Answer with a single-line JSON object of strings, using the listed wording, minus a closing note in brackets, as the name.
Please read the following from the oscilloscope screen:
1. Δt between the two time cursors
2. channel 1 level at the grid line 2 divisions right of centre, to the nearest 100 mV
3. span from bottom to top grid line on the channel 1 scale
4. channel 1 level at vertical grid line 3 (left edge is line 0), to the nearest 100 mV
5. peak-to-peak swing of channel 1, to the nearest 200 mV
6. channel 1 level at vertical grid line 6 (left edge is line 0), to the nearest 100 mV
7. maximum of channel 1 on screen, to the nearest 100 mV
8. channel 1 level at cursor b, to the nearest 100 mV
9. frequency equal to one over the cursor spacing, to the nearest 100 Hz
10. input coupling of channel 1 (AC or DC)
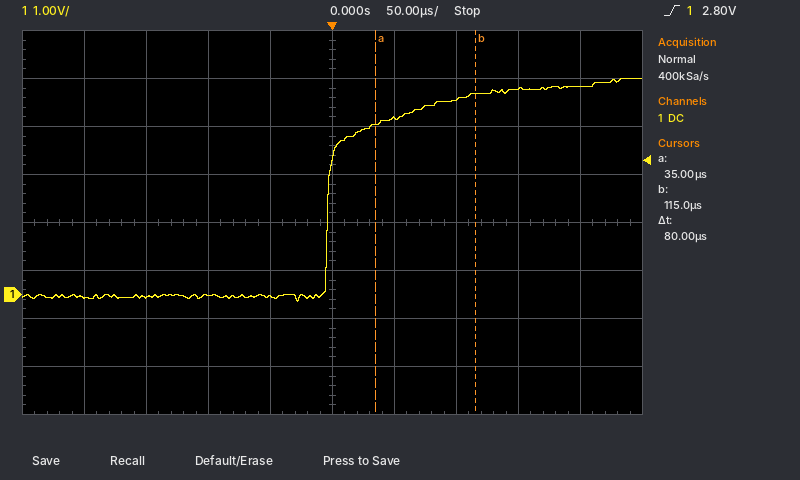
{"Δt between the two time cursors": "80 µs", "channel 1 level at the grid line 2 divisions right of centre, to the nearest 100 mV": "4.1 V", "span from bottom to top grid line on the channel 1 scale": "8 V", "channel 1 level at vertical grid line 3 (left edge is line 0), to the nearest 100 mV": "0.0 V", "peak-to-peak swing of channel 1, to the nearest 200 mV": "4.6 V", "channel 1 level at vertical grid line 6 (left edge is line 0), to the nearest 100 mV": "3.7 V", "maximum of channel 1 on screen, to the nearest 100 mV": "4.5 V", "channel 1 level at cursor b, to the nearest 100 mV": "4.2 V", "frequency equal to one over the cursor spacing, to the nearest 100 Hz": "12.5 kHz", "input coupling of channel 1": "DC"}
